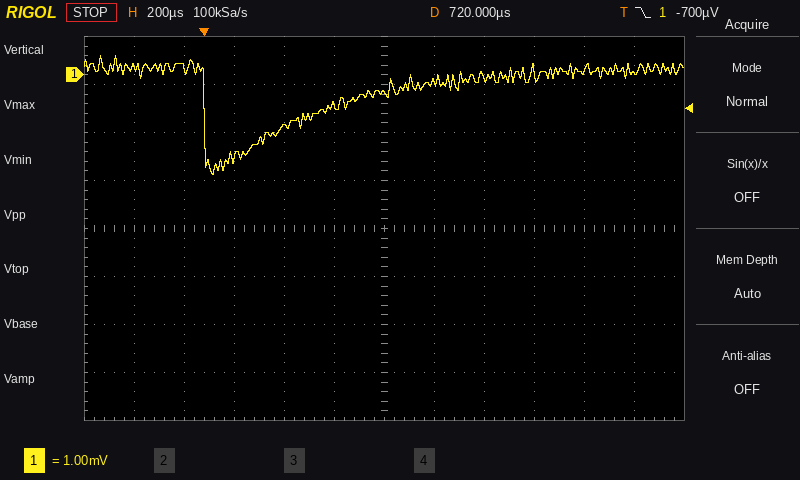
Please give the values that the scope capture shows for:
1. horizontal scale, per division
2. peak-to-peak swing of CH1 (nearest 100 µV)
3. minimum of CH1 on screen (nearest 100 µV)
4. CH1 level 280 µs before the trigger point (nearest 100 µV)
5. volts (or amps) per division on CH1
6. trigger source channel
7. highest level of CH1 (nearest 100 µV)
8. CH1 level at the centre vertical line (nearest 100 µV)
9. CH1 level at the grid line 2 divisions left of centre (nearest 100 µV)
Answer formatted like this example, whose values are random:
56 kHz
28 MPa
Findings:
200 µs
2.5 mV
-2.1 mV
200 µV
1 mV
CH1
400 µV
-400 µV
-1.1 mV
